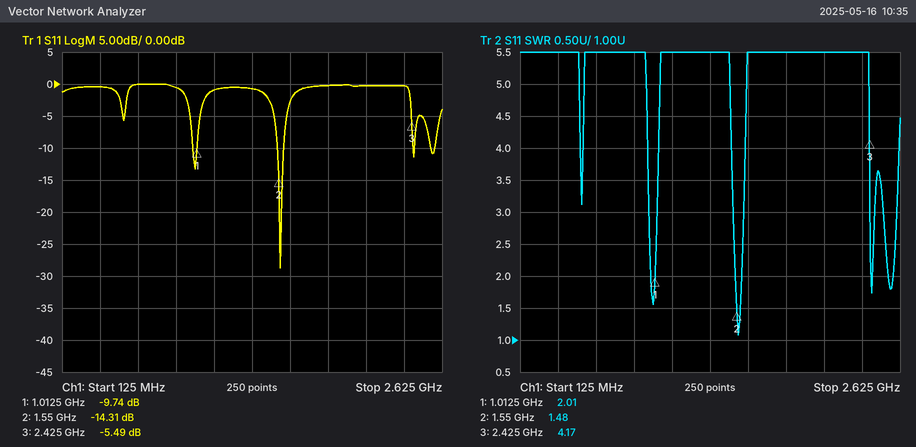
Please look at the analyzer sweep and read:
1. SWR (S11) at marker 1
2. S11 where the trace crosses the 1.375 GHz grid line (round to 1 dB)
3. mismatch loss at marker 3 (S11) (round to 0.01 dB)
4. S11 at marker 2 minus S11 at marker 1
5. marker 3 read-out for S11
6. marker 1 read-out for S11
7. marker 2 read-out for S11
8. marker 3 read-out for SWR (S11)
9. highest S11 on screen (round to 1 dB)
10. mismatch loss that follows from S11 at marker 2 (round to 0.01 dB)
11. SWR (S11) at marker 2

2.01
-1 dB
1.44 dB
-4.57 dB
-5.49 dB
-9.74 dB
-14.31 dB
4.17
0 dB
0.16 dB
1.48
